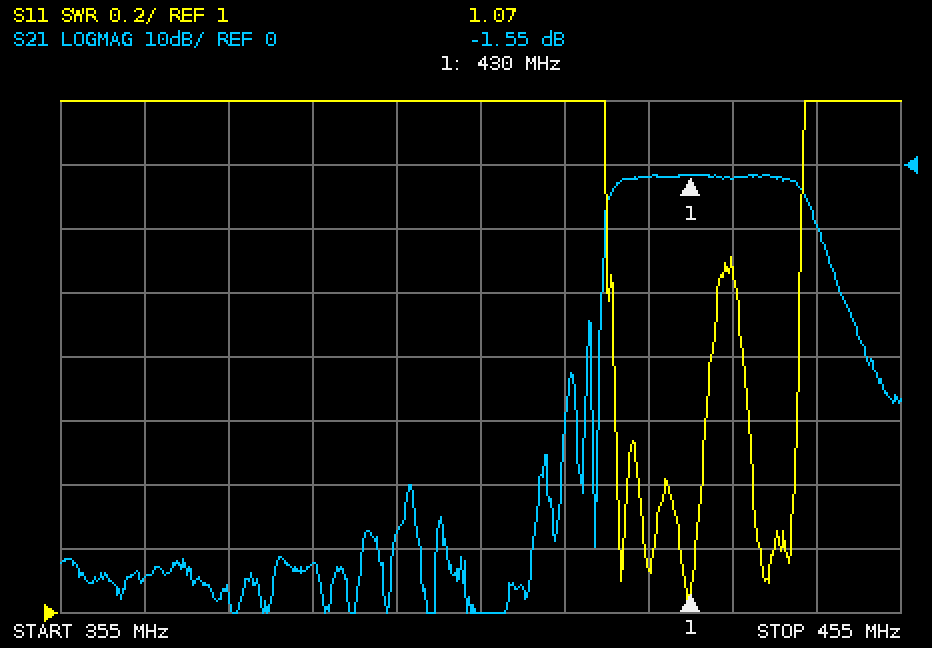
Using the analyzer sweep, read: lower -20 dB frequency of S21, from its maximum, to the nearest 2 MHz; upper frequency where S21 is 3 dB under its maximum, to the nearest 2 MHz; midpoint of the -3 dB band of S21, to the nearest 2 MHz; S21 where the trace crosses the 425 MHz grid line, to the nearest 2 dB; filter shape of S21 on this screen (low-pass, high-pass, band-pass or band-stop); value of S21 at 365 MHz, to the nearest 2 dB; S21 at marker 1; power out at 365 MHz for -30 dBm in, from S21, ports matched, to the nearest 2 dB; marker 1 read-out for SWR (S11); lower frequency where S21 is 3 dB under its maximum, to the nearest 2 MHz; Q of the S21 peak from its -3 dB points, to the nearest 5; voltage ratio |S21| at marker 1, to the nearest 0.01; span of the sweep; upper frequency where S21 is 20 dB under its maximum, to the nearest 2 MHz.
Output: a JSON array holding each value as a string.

["420 MHz", "444 MHz", "432 MHz", "-2 dB", "band-pass", "-64 dB", "-1.55 dB", "-94 dBm", "1.07", "420 MHz", "20", "0.84", "100 MHz", "448 MHz"]
